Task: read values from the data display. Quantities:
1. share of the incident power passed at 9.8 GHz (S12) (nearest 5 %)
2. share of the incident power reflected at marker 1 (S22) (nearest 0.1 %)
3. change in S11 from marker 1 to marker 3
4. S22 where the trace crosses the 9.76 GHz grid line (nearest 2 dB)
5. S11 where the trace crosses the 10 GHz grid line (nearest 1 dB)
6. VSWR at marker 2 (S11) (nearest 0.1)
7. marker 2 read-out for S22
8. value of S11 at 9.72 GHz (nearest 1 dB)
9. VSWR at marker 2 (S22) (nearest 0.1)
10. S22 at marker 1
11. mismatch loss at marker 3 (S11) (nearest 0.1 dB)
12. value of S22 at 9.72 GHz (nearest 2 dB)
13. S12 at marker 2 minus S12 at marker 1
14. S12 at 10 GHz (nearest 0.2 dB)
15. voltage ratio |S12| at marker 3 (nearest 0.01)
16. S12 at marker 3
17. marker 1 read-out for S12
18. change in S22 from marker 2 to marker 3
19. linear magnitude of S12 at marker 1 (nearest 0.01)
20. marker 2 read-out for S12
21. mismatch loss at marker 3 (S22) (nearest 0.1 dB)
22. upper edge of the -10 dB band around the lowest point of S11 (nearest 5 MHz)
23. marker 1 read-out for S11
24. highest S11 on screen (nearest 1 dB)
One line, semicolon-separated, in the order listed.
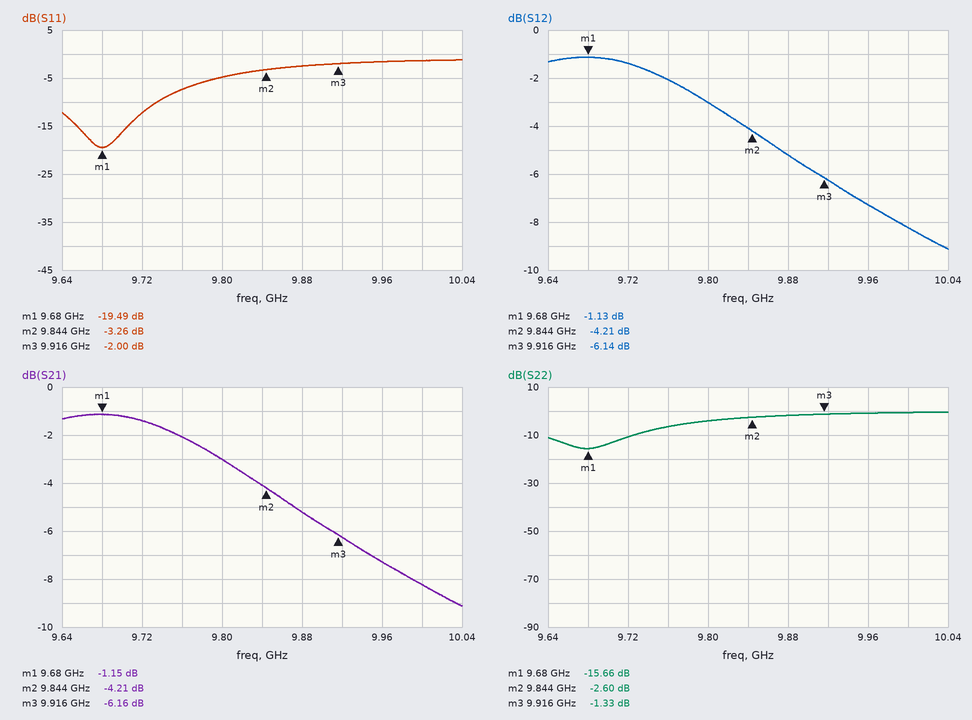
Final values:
50 %; 2.7 %; 17.49 dB; -6 dB; -1 dB; 5.4; -2.60 dB; -12 dB; 6.7; -15.66 dB; 4.3 dB; -10 dB; -3.08 dB; -8.2 dB; 0.49; -6.14 dB; -1.13 dB; 1.27 dB; 0.88; -4.21 dB; 5.8 dB; 9.735 GHz; -19.49 dB; -1 dB
